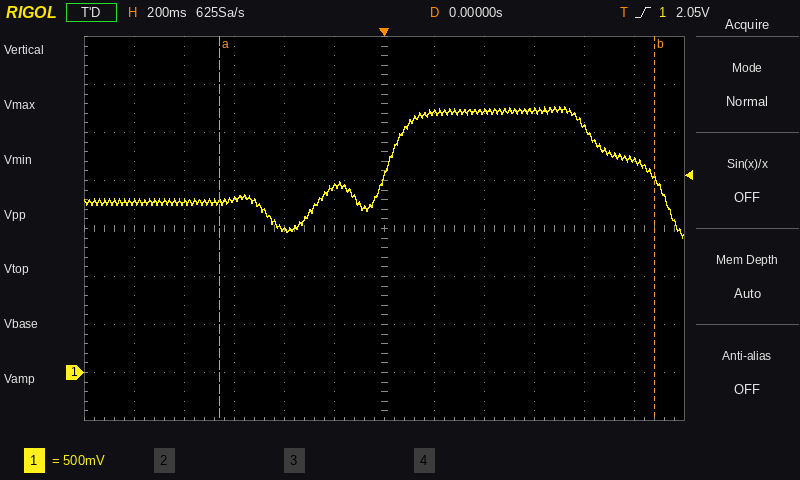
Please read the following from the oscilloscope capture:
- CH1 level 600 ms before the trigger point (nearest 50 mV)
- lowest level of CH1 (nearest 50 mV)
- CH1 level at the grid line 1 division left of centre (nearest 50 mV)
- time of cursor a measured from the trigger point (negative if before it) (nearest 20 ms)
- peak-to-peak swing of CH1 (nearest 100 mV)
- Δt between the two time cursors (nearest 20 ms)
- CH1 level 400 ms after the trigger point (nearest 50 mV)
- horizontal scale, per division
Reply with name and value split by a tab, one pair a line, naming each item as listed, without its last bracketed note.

CH1 level 600 ms before the trigger point	1.80 V
lowest level of CH1	1.40 V
CH1 level at the grid line 1 division left of centre	1.95 V
time of cursor a measured from the trigger point (negative if before it)	-660 ms
peak-to-peak swing of CH1	1.40 V
Δt between the two time cursors	1.74 s
CH1 level 400 ms after the trigger point	2.70 V
horizontal scale, per division	200 ms
